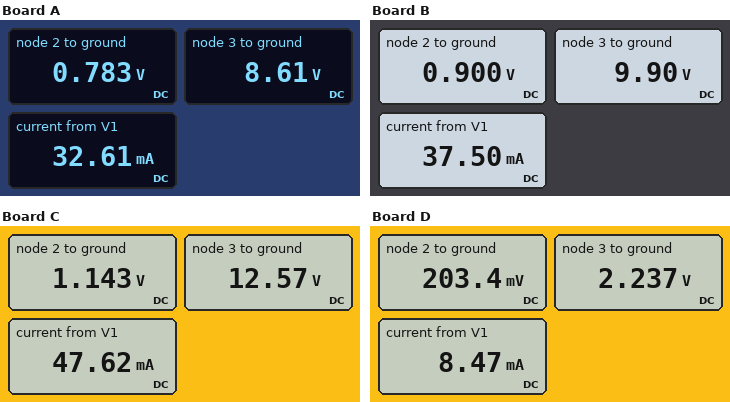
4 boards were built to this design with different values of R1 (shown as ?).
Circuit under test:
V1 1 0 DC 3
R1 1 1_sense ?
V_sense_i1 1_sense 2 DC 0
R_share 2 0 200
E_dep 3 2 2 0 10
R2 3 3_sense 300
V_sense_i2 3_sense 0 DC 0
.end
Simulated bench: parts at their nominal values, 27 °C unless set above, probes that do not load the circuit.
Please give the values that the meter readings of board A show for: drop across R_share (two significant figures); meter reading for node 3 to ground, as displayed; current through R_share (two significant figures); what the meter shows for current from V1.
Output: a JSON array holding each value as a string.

["780 mV", "8.61 V", "3.9 mA", "32.61 mA"]
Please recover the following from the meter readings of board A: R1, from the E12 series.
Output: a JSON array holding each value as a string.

["68 Ω"]
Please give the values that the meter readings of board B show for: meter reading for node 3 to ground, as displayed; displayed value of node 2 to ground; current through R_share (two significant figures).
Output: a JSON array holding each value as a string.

["9.90 V", "0.900 V", "4.5 mA"]
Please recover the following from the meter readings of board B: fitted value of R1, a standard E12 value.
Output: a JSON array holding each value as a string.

["56 Ω"]
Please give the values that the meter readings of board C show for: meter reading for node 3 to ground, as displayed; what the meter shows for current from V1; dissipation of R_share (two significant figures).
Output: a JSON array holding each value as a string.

["12.57 V", "47.62 mA", "6.5 mW"]
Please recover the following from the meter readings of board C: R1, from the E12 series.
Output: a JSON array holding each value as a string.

["39 Ω"]
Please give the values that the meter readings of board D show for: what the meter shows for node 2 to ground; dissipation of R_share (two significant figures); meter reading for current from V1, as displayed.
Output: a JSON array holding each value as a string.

["203.4 mV", "210 µW", "8.47 mA"]
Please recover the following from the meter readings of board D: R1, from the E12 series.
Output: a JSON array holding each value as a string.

["330 Ω"]
